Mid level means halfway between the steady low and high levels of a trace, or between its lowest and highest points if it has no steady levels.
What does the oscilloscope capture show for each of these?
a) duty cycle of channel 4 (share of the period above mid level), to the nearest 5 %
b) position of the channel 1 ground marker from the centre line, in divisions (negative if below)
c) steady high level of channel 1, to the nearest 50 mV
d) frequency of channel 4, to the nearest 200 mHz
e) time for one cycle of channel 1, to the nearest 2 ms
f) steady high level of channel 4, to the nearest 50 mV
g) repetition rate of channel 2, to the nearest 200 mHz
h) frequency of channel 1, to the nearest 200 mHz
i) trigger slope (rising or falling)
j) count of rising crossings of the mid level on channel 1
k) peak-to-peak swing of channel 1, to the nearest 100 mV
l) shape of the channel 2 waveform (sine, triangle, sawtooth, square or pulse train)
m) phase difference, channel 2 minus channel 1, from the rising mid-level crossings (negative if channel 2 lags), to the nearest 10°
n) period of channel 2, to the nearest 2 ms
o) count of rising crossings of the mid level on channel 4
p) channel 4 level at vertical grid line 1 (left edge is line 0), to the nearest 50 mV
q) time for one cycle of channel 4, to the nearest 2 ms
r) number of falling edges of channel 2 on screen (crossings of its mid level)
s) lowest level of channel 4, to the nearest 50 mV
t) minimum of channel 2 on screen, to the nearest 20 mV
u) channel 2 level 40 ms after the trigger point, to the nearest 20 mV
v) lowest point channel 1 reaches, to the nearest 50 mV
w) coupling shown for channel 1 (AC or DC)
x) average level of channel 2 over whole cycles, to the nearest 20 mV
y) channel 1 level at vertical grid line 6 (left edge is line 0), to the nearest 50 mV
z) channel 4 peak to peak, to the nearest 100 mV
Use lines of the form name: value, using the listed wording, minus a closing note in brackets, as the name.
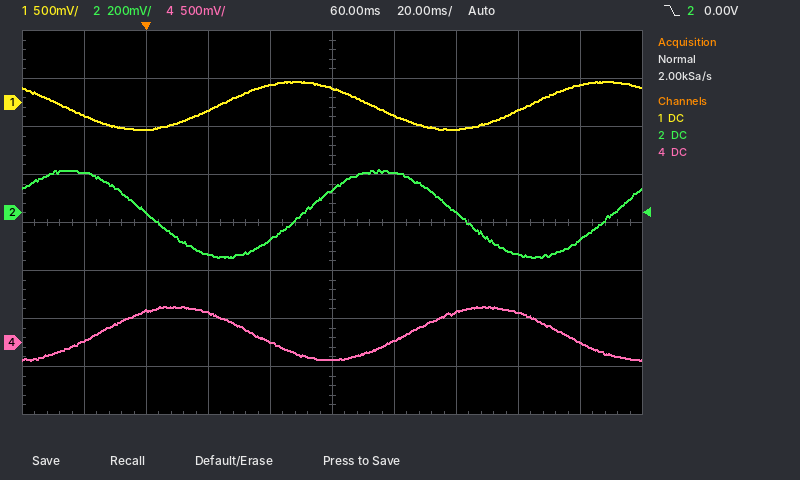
duty cycle of channel 4 (share of the period above mid level), to the nearest 5 %: 50 %
position of the channel 1 ground marker from the centre line, in divisions: +2.5 div
steady high level of channel 1, to the nearest 50 mV: 200 mV
frequency of channel 4, to the nearest 200 mHz: 10.0 Hz
time for one cycle of channel 1, to the nearest 2 ms: 100 ms
steady high level of channel 4, to the nearest 50 mV: 350 mV
repetition rate of channel 2, to the nearest 200 mHz: 10.0 Hz
frequency of channel 1, to the nearest 200 mHz: 10.0 Hz
trigger slope: falling
count of rising crossings of the mid level on channel 1: 2
peak-to-peak swing of channel 1, to the nearest 100 mV: 500 mV
shape of the channel 2 waveform: sine
phase difference, channel 2 minus channel 1, from the rising mid-level crossings (negative if channel 2 lags), to the nearest 10°: -100°
period of channel 2, to the nearest 2 ms: 100 ms
count of rising crossings of the mid level on channel 4: 2
channel 4 level at vertical grid line 1 (left edge is line 0), to the nearest 50 mV: 0 mV
time for one cycle of channel 4, to the nearest 2 ms: 100 ms
number of falling edges of channel 2 on screen: 2
lowest level of channel 4, to the nearest 50 mV: -200 mV
minimum of channel 2 on screen, to the nearest 20 mV: -180 mV
channel 2 level 40 ms after the trigger point, to the nearest 20 mV: -120 mV
lowest point channel 1 reaches, to the nearest 50 mV: -300 mV
coupling shown for channel 1: DC
average level of channel 2 over whole cycles, to the nearest 20 mV: 0 mV
channel 1 level at vertical grid line 6 (left edge is line 0), to the nearest 50 mV: -150 mV
channel 4 peak to peak, to the nearest 100 mV: 600 mV
